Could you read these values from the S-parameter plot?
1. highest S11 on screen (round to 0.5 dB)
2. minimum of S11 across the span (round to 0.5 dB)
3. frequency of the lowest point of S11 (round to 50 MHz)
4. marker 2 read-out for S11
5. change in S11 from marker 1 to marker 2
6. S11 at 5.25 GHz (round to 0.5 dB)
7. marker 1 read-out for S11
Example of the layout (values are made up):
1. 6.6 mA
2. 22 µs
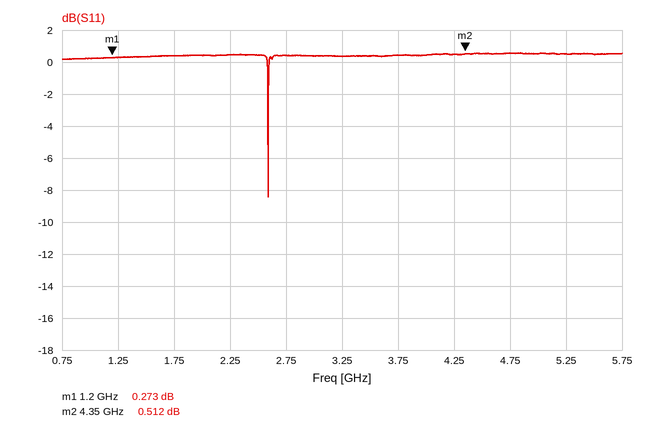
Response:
1. 0.5 dB
2. -8.5 dB
3. 2.60 GHz
4. 0.512 dB
5. 0.239 dB
6. 0.5 dB
7. 0.273 dB
